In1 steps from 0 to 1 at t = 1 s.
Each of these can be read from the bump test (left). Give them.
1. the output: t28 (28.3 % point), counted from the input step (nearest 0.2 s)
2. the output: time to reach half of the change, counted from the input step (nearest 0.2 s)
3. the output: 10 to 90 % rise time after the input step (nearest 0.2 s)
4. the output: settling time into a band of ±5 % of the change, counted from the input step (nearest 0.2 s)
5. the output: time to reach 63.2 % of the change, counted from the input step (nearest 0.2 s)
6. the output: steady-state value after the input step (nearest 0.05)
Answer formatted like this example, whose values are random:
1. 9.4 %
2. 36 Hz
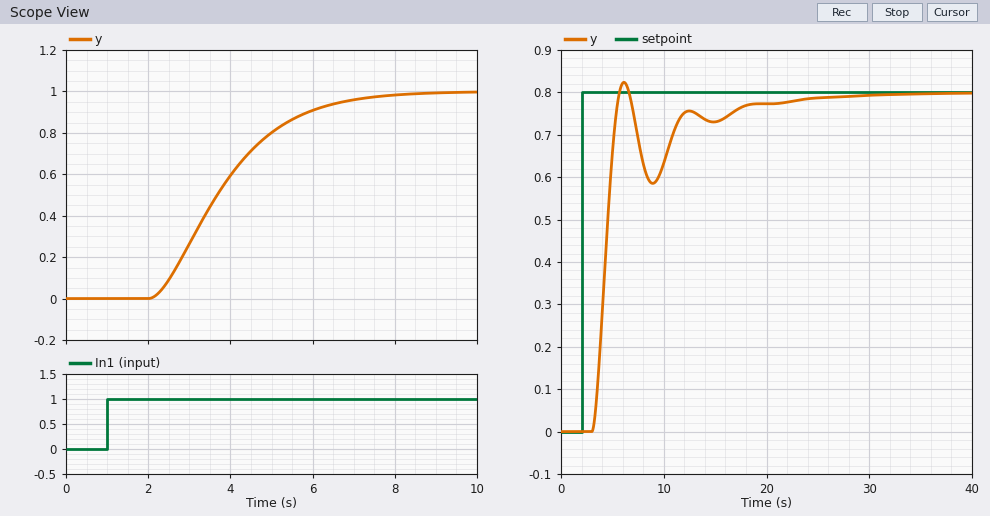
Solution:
1. 2.0 s
2. 2.6 s
3. 3.4 s
4. 5.8 s
5. 3.2 s
6. 1.00
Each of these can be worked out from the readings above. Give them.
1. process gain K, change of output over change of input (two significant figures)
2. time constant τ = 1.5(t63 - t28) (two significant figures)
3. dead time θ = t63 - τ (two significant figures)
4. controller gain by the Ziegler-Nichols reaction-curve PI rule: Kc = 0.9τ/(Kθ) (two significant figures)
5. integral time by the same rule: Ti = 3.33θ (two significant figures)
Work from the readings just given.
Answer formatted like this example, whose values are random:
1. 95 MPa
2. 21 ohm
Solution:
1. 1.0
2. 1.8 s
3. 1.4 s
4. 1.2
5. 4.7 s
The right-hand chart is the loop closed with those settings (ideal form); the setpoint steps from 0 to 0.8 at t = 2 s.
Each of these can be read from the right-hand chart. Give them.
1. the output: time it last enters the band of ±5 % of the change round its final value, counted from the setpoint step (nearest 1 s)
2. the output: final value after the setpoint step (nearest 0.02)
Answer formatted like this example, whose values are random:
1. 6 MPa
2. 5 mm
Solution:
1. 15 s
2. 0.80
